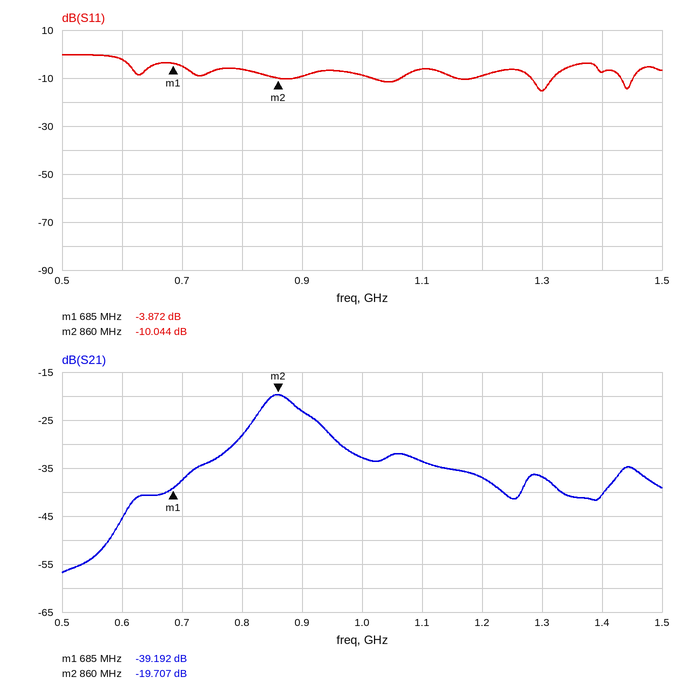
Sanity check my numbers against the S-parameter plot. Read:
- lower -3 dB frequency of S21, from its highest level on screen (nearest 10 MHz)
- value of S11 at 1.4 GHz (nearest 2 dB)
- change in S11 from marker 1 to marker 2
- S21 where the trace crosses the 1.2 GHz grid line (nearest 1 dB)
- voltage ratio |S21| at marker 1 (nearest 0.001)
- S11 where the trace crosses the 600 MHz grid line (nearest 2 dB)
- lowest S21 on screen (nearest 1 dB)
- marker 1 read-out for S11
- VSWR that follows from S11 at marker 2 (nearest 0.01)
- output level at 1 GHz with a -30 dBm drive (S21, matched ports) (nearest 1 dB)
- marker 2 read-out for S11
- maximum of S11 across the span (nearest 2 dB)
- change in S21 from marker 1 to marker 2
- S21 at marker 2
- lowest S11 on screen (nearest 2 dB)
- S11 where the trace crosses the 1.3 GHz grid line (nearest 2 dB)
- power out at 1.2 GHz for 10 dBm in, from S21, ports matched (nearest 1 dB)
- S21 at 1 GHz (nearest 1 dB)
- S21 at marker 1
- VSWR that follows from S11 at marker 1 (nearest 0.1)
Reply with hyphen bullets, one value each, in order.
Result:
- 830 MHz
- -8 dB
- -6.172 dB
- -37 dB
- 0.011
- -2 dB
- -57 dB
- -3.872 dB
- 1.92
- -63 dBm
- -10.044 dB
- 0 dB
- 19.485 dB
- -19.707 dB
- -16 dB
- -16 dB
- -27 dBm
- -33 dB
- -39.192 dB
- 4.6
